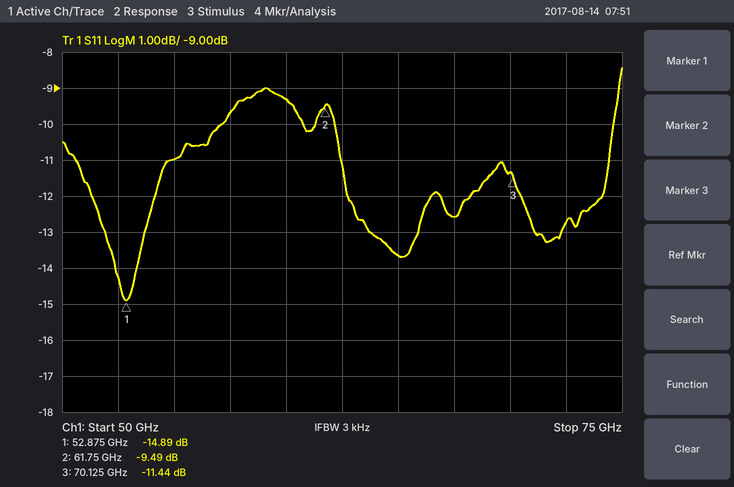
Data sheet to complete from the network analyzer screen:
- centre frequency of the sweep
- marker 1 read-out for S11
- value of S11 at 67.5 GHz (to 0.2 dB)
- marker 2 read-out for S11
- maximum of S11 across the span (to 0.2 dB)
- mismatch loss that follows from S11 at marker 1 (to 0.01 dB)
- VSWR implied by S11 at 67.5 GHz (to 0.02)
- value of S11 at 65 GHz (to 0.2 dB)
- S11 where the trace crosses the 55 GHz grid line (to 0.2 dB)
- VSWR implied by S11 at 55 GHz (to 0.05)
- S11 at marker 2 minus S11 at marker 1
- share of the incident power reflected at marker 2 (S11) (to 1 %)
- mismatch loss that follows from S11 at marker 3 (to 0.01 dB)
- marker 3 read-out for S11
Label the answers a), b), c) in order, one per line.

a) 62.5 GHz
b) -14.89 dB
c) -12.6 dB
d) -9.49 dB
e) -8.4 dB
f) 0.14 dB
g) 1.62
h) -13.6 dB
i) -11.0 dB
j) 1.80
k) 5.40 dB
l) 11 %
m) 0.32 dB
n) -11.44 dB
